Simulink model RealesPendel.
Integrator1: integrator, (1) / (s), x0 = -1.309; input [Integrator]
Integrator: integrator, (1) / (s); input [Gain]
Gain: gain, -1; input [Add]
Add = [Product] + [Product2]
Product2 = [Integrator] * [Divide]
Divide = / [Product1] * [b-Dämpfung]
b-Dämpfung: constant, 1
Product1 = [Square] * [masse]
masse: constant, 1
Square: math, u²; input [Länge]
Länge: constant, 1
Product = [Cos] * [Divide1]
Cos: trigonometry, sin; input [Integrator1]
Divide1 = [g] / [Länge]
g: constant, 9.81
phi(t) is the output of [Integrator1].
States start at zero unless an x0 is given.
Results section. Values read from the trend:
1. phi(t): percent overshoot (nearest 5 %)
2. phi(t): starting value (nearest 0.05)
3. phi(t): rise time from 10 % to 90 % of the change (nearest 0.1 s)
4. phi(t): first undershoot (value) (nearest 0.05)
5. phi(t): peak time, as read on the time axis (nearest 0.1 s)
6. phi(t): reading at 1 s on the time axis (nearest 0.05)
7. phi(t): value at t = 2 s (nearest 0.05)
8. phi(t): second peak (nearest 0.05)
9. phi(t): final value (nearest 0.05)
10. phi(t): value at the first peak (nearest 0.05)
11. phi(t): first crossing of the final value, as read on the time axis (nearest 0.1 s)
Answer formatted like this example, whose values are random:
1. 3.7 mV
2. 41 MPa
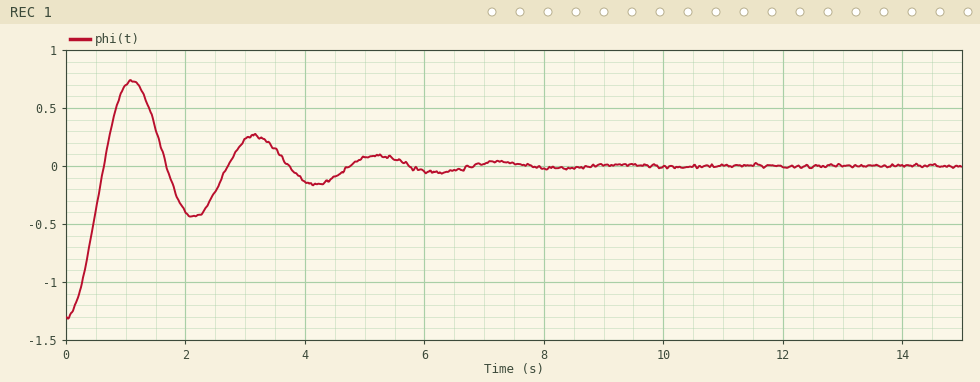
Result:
1. 55 %
2. -1.30
3. 0.4 s
4. -0.45
5. 1.1 s
6. 0.70
7. -0.40
8. 0.25
9. 0.00
10. 0.75
11. 0.6 s
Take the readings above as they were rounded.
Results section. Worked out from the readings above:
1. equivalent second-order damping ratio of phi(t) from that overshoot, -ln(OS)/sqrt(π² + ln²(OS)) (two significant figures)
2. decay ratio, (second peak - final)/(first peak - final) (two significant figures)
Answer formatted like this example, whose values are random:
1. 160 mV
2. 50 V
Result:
1. 0.19
2. 0.33
